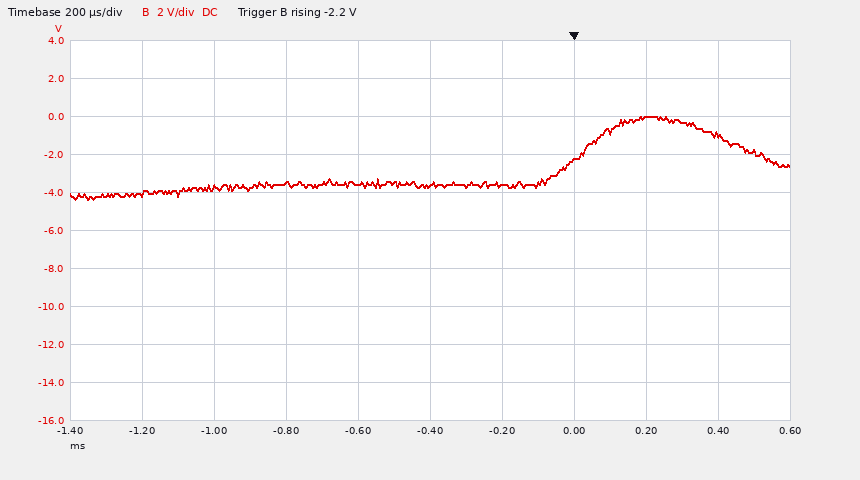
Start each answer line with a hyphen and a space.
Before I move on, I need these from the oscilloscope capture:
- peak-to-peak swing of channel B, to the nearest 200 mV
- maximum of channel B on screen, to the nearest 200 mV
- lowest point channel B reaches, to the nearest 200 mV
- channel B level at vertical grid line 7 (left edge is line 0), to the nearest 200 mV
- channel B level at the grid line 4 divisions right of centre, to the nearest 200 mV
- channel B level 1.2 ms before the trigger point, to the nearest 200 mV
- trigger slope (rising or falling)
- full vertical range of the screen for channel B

- 4.4 V
- 0.0 V
- -4.4 V
- -2.2 V
- -1.0 V
- -4.0 V
- rising
- 20 V
